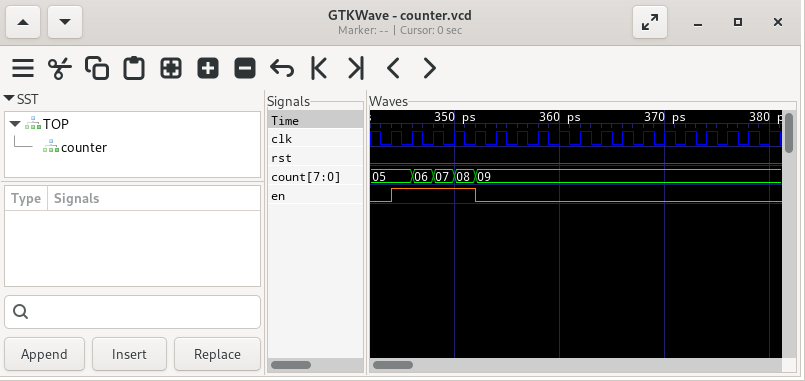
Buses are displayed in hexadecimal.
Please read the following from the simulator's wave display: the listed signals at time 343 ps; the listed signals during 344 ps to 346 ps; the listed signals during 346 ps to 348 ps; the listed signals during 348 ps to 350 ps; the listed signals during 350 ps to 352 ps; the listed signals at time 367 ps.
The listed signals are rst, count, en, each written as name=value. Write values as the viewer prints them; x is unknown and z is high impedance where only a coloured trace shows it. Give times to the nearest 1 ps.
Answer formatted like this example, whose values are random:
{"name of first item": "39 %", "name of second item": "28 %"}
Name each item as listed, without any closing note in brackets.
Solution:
{"the listed signals at time 343 ps": "rst=0, count=05, en=0", "the listed signals during 344 ps to 346 ps": "rst=0, count=05, en=1", "the listed signals during 346 ps to 348 ps": "rst=0, count=06, en=1", "the listed signals during 348 ps to 350 ps": "rst=0, count=07, en=1", "the listed signals during 350 ps to 352 ps": "rst=0, count=08, en=1", "the listed signals at time 367 ps": "rst=0, count=09, en=0"}
